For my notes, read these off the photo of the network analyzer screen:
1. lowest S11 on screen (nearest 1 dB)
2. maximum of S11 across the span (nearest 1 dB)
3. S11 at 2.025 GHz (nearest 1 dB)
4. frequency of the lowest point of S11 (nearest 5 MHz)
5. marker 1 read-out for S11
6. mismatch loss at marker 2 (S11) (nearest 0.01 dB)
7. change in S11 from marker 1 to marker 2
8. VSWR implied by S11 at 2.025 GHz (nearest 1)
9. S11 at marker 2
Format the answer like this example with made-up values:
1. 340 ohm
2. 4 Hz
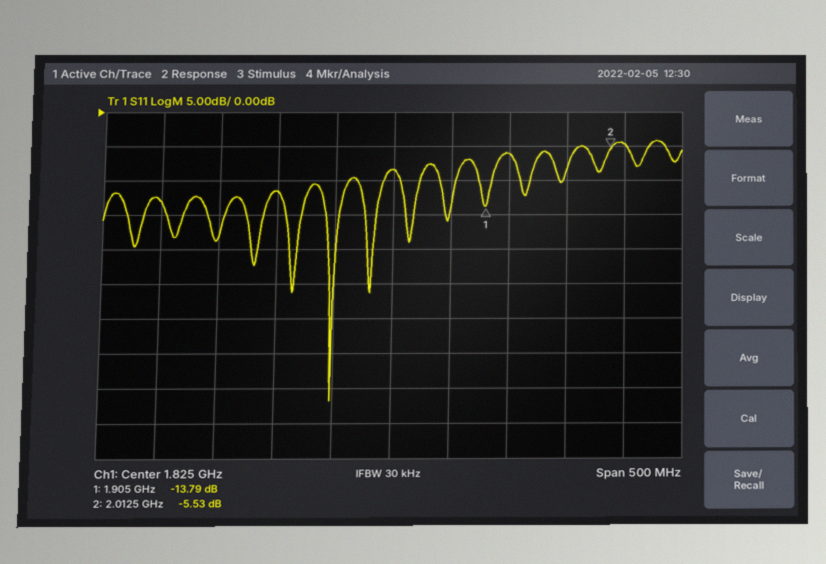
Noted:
1. -42 dB
2. -4 dB
3. -5 dB
4. 1.775 GHz
5. -13.79 dB
6. 1.43 dB
7. 8.26 dB
8. 4
9. -5.53 dB
